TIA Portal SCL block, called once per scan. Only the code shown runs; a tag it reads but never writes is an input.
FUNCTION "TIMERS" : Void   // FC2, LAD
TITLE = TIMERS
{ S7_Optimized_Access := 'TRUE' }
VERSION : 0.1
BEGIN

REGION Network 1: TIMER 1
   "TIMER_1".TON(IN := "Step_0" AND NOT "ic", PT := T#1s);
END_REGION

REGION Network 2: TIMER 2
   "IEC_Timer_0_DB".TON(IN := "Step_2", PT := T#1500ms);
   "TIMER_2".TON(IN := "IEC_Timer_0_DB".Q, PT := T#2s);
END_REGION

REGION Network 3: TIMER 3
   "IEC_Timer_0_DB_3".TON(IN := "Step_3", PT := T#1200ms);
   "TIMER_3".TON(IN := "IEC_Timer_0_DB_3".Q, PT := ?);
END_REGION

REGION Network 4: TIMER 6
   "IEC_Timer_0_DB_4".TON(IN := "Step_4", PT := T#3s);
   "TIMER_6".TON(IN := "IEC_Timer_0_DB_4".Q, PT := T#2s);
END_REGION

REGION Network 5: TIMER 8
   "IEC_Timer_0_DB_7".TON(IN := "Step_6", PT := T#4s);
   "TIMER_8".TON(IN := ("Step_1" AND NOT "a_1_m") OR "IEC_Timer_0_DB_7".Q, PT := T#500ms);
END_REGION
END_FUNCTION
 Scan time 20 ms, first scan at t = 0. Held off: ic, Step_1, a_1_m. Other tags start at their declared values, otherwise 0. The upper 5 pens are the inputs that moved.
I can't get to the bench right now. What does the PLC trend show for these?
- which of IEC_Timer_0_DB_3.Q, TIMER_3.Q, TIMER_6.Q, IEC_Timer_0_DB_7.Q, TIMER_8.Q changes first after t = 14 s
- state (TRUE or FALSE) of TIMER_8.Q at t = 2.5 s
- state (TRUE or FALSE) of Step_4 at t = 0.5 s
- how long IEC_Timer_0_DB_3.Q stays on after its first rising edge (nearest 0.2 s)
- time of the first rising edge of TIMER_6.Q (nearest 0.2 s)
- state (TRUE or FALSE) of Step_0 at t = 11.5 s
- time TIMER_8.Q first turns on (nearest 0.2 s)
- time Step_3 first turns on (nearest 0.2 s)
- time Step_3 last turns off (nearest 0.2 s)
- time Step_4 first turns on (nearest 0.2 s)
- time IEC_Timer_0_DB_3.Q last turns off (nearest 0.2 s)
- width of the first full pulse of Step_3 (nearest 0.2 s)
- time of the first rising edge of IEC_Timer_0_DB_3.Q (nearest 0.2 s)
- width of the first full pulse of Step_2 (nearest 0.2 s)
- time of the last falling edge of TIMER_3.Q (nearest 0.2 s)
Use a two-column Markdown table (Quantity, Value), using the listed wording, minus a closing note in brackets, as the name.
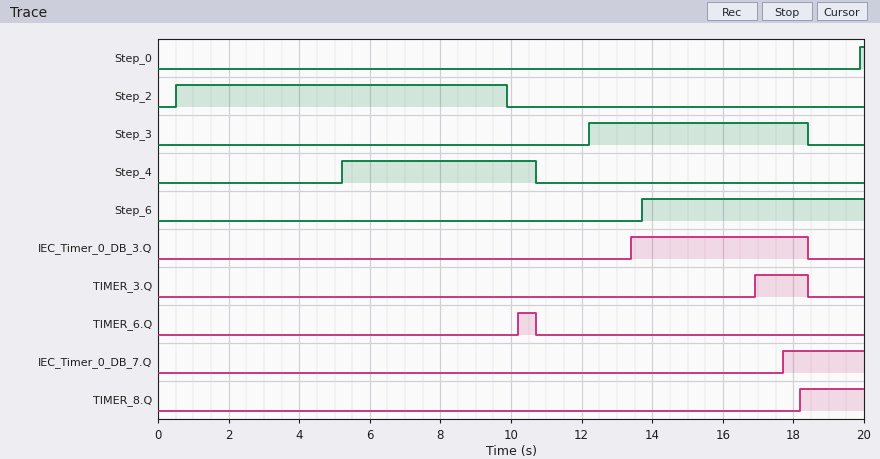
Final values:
| Quantity | Value |
|---|---|
| which of IEC_Timer_0_DB_3.Q, TIMER_3.Q, TIMER_6.Q, IEC_Timer_0_DB_7.Q, TIMER_8.Q changes first after t = 14 s | TIMER_3.Q |
| state (TRUE or FALSE) of TIMER_8.Q at t = 2.5 s | FALSE |
| state (TRUE or FALSE) of Step_4 at t = 0.5 s | FALSE |
| how long IEC_Timer_0_DB_3.Q stays on after its first rising edge | 5.0 s |
| time of the first rising edge of TIMER_6.Q | 10.2 s |
| state (TRUE or FALSE) of Step_0 at t = 11.5 s | FALSE |
| time TIMER_8.Q first turns on | 18.2 s |
| time Step_3 first turns on | 12.2 s |
| time Step_3 last turns off | 18.4 s |
| time Step_4 first turns on | 5.2 s |
| time IEC_Timer_0_DB_3.Q last turns off | 18.4 s |
| width of the first full pulse of Step_3 | 6.2 s |
| time of the first rising edge of IEC_Timer_0_DB_3.Q | 13.4 s |
| width of the first full pulse of Step_2 | 9.4 s |
| time of the last falling edge of TIMER_3.Q | 18.4 s |
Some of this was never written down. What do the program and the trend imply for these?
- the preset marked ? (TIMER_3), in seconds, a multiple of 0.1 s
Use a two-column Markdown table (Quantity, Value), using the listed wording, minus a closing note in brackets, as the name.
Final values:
| Quantity | Value |
|---|---|
| the preset marked ? (TIMER_3), in seconds, a multiple of 0.1 s | 3.5 s |
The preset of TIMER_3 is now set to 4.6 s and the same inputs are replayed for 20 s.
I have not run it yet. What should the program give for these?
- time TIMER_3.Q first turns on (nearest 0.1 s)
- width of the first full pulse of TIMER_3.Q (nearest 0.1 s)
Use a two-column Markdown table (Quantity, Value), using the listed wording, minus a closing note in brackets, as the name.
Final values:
| Quantity | Value |
|---|---|
| time TIMER_3.Q first turns on | 18.0 s |
| width of the first full pulse of TIMER_3.Q | 0.4 s |
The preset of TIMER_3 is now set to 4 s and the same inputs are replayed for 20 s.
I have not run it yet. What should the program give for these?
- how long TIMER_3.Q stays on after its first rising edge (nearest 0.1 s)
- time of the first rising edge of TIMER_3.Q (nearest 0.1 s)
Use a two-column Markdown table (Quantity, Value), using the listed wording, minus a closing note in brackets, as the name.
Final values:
| Quantity | Value |
|---|---|
| how long TIMER_3.Q stays on after its first rising edge | 1.0 s |
| time of the first rising edge of TIMER_3.Q | 17.4 s |
